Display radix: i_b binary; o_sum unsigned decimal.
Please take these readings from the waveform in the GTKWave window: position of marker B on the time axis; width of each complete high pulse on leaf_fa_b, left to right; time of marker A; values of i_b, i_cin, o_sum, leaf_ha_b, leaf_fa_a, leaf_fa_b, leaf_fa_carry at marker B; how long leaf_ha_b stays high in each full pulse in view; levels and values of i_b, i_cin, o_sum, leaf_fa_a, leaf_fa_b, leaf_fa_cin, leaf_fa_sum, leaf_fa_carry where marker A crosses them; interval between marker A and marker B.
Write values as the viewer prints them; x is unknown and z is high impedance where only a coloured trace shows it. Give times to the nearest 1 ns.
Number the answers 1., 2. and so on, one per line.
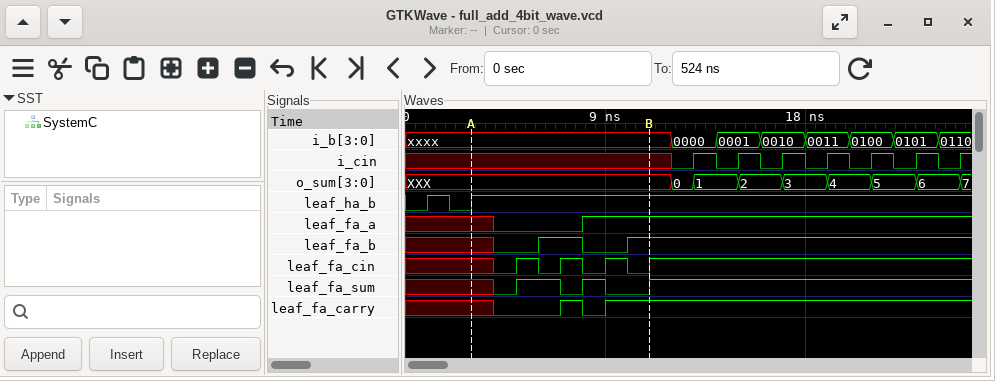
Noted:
1. 11 ns
2. 2 ns
3. 3 ns
4. i_b=xxxx, i_cin=x, o_sum=XXX, leaf_ha_b=1, leaf_fa_a=1, leaf_fa_b=1, leaf_fa_carry=1
5. 1 ns
6. i_b=xxxx, i_cin=x, o_sum=XXX, leaf_fa_a=x, leaf_fa_b=x, leaf_fa_cin=x, leaf_fa_sum=x, leaf_fa_carry=x
7. 8 ns
